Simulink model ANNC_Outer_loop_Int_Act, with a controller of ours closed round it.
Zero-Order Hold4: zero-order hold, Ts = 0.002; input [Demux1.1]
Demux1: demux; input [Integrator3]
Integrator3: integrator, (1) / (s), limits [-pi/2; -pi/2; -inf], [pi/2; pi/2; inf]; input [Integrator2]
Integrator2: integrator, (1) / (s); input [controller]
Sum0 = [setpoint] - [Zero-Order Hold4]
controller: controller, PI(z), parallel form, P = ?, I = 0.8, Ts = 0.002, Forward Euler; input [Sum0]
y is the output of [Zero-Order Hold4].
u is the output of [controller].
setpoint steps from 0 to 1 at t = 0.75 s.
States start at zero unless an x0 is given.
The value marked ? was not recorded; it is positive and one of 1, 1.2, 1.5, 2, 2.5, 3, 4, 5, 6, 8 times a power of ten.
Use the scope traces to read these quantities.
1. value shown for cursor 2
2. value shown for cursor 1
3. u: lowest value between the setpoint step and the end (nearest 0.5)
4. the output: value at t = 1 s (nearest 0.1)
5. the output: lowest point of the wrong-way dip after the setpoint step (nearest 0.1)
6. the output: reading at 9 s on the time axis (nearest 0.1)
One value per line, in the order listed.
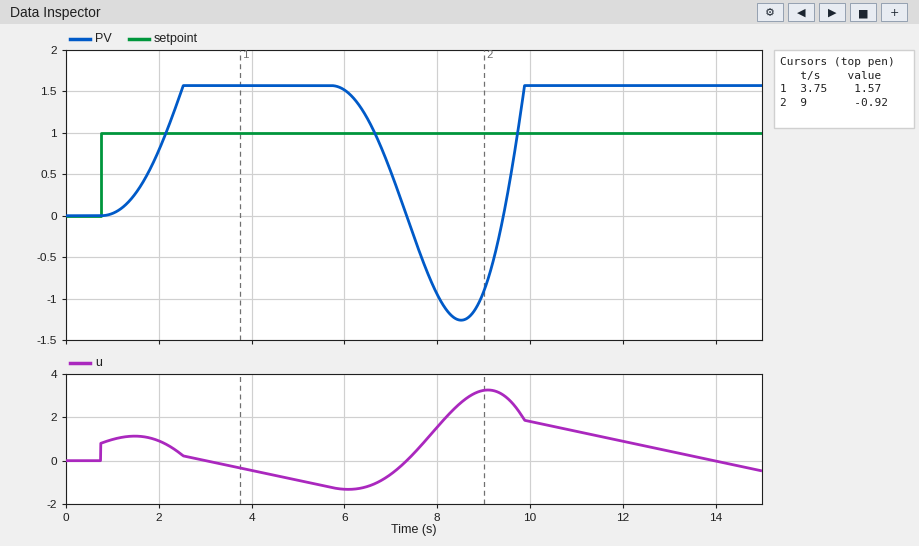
-0.92
1.57
-1.5
0.0
-1.3
-0.9
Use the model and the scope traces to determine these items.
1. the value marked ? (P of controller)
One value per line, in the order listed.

0.8
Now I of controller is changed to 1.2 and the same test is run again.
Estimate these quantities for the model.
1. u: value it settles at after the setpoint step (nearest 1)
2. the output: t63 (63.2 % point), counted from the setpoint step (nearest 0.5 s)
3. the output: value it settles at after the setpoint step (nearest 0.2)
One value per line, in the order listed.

0
1.5 s
1.6
